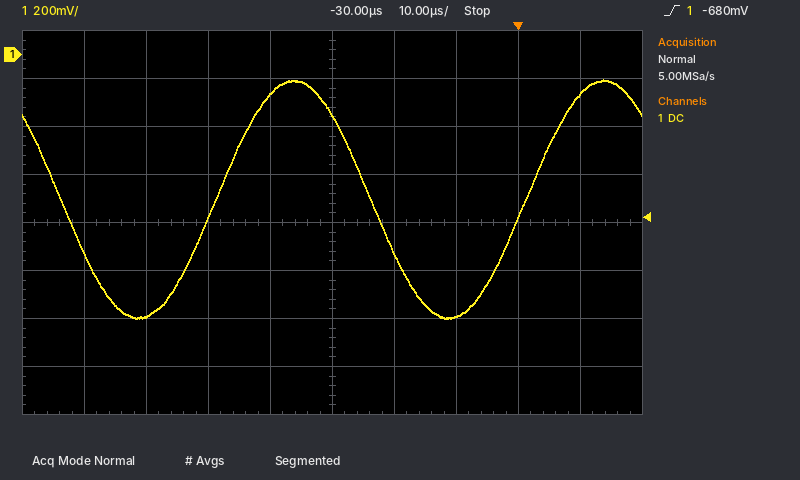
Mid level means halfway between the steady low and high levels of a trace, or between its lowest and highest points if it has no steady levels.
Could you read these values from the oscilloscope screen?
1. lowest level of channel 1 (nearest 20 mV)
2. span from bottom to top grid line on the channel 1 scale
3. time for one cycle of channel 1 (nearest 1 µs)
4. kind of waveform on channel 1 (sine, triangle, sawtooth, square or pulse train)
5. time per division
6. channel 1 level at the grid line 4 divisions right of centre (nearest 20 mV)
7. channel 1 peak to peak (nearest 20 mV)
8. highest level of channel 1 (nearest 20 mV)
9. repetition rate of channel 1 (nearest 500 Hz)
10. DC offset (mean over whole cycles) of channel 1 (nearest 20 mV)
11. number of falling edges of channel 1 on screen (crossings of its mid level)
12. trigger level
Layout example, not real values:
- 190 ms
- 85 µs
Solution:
- -1.10 V
- 1.6 V
- 50 µs
- sine
- 10 µs
- -160 mV
- 1.00 V
- -100 mV
- 20.0 kHz
- -600 mV
- 2
- -680 mV
